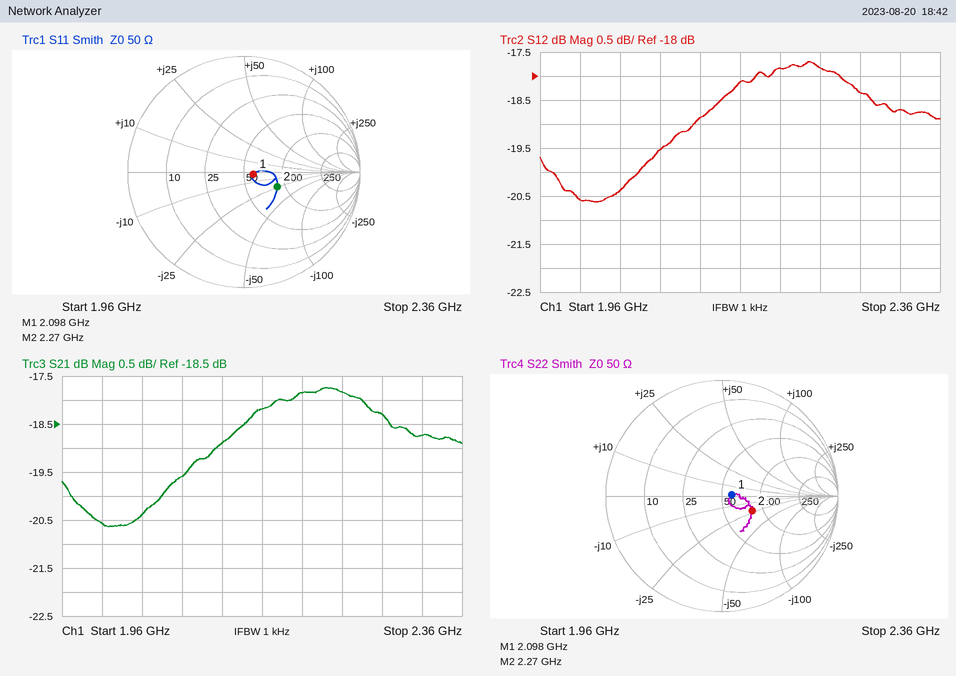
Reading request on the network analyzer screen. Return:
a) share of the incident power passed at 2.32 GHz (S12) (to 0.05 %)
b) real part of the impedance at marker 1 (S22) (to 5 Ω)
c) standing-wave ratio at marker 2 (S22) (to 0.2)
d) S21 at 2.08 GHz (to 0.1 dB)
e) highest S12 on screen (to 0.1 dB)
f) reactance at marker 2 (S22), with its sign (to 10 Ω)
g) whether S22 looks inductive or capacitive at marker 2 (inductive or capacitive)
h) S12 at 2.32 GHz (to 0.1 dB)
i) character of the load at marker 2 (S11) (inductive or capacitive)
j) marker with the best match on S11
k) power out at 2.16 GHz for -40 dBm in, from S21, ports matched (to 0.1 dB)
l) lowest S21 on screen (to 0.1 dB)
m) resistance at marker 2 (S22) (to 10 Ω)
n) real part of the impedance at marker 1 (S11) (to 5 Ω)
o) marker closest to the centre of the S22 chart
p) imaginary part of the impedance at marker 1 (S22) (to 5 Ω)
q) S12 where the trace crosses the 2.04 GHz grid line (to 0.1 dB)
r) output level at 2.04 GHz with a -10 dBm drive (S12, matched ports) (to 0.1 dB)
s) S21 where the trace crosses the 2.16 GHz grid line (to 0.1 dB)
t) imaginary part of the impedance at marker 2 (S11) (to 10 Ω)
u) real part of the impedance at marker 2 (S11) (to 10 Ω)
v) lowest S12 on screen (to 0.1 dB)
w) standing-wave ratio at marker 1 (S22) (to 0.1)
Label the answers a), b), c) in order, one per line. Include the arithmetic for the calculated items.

a) 10^(-18.7/10) ≈ 1.35 %
b) 60 Ω
c) 1.8
d) -19.6 dB
e) -17.7 dB
f) -20 Ω
g) capacitive
h) -18.7 dB
i) capacitive
j) marker 1
k) -40 dBm + (-18.2 dB) = -58.2 dBm
l) -20.6 dB
m) 80 Ω
n) 60 Ω
o) marker 1
p) 0 Ω
q) -20.4 dB
r) -10 dBm + (-20.4 dB) = -30.4 dBm
s) -18.2 dB
t) -20 Ω
u) 90 Ω
v) -20.6 dB
w) 1.2
